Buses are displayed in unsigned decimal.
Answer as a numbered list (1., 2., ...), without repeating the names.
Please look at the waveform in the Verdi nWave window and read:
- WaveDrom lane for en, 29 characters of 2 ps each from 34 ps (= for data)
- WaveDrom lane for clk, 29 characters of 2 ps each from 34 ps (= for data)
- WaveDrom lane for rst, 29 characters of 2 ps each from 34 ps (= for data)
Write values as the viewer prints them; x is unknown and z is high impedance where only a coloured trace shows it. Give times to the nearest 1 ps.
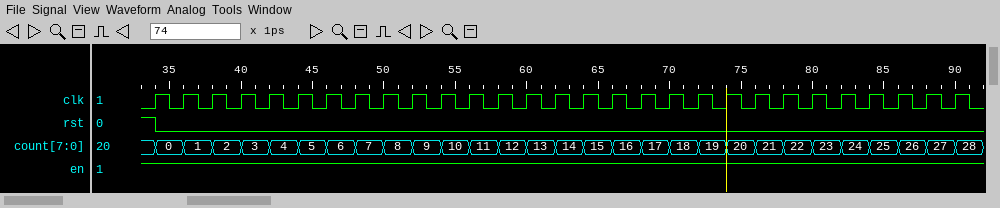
1. {name: 'en', wave: '1............................'}
2. {name: 'clk', wave: 'p............................'}
3. {name: 'rst', wave: '0............................'}
